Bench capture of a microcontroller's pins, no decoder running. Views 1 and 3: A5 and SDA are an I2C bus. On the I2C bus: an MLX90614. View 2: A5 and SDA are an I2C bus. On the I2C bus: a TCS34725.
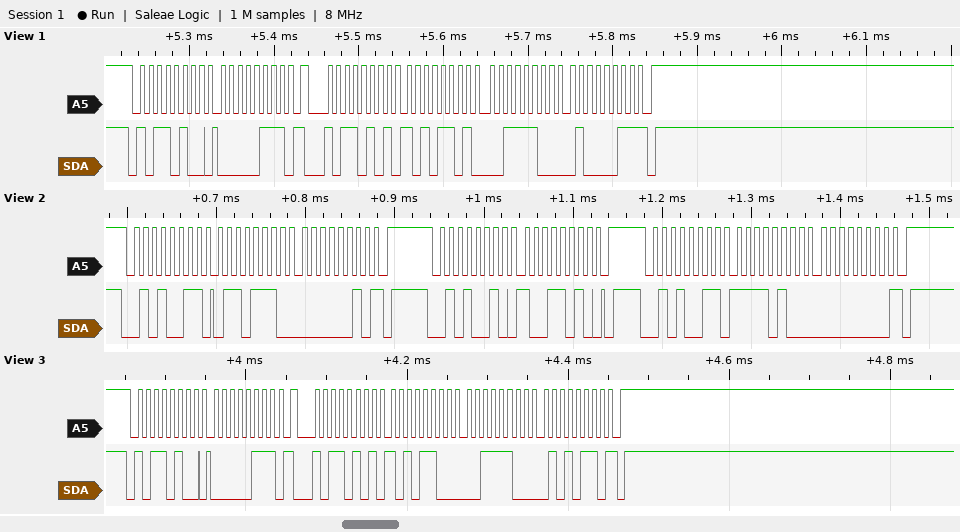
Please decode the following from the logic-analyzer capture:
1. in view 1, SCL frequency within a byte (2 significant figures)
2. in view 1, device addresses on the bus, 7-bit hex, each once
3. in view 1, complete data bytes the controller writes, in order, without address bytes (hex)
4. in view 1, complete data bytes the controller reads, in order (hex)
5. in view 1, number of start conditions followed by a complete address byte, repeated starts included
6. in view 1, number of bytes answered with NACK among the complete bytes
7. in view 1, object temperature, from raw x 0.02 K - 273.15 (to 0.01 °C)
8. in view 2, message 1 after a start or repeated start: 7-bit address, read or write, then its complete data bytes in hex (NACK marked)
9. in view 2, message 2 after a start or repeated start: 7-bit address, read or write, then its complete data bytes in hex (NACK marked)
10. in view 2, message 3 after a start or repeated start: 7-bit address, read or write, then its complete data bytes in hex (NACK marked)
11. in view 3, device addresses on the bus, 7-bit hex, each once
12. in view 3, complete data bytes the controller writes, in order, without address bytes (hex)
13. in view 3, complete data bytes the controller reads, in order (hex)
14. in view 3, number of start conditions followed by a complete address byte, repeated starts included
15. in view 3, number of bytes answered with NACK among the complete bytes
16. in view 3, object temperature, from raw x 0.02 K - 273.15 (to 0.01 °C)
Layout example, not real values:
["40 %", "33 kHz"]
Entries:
["100 kHz", "0x5A", "07", "AD 3C 43", "2", "1", "37.51 °C", "0x29 read: 6E 02 NACK", "0x29 write: 9A", "0x29 read: F4 00 NACK", "0x5A", "07", "AC 3C 56", "2", "1", "37.49 °C"]
